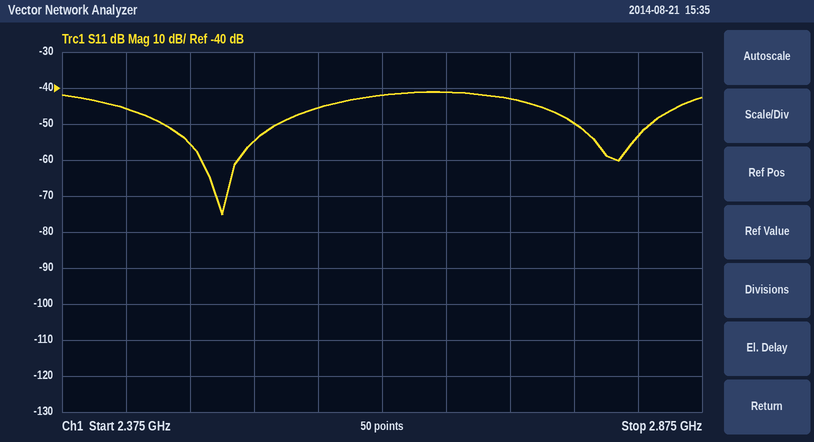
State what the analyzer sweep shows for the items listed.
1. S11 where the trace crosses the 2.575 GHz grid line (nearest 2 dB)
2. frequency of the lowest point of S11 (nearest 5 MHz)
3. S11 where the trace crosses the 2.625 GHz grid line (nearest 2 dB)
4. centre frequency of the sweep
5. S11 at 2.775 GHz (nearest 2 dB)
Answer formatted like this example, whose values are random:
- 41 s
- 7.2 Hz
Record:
- -46 dB
- 2.500 GHz
- -42 dB
- 2.625 GHz
- -50 dB
